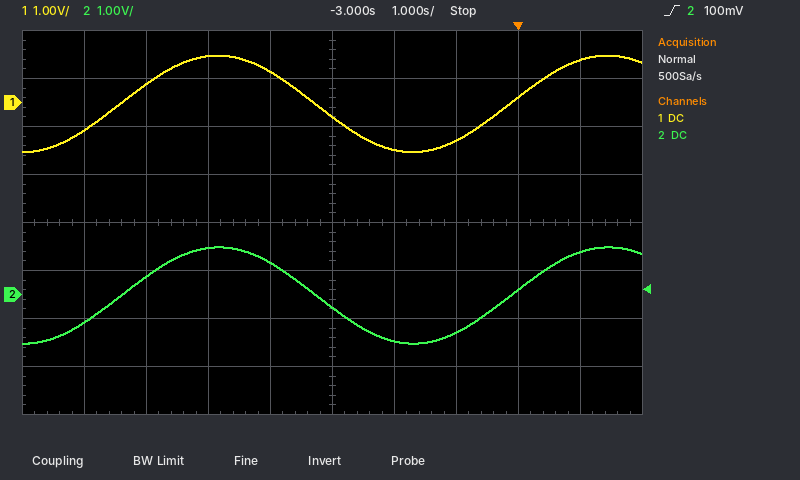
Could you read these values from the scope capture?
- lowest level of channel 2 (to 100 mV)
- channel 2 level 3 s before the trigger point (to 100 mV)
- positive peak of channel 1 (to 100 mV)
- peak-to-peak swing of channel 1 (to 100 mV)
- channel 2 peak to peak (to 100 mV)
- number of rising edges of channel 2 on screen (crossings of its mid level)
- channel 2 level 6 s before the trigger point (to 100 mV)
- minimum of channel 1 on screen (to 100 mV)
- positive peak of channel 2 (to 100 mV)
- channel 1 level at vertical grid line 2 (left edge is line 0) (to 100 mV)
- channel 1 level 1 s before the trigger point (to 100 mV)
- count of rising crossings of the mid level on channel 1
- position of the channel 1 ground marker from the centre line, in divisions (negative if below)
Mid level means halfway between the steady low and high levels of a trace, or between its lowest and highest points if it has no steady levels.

-1.0 V
-300 mV
1.0 V
2.0 V
2.0 V
2
400 mV
-1.0 V
1.0 V
400 mV
-800 mV
2
+2.5 div
